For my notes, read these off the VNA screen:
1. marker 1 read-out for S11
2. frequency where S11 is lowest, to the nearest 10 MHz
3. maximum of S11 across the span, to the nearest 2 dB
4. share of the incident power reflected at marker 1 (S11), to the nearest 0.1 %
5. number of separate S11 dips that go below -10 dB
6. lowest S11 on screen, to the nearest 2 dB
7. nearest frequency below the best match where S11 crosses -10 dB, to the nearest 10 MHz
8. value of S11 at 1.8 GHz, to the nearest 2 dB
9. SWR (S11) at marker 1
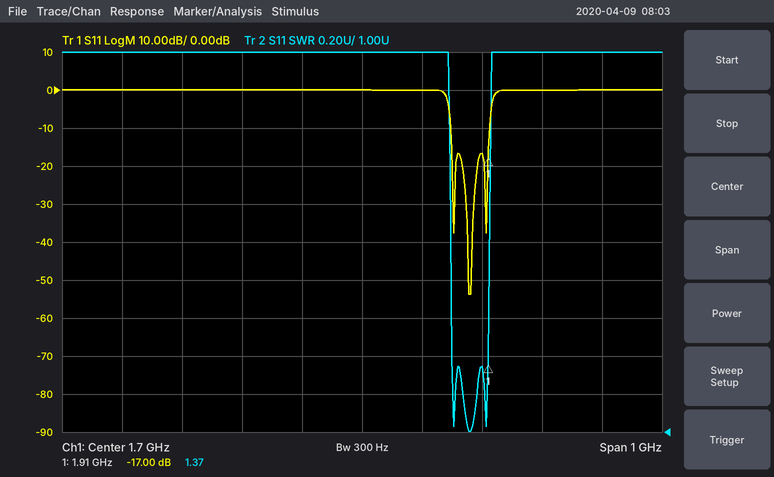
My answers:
-17.00 dB
1.88 GHz
0 dB
2.0 %
3
-54 dB
1.85 GHz
0 dB
1.37
